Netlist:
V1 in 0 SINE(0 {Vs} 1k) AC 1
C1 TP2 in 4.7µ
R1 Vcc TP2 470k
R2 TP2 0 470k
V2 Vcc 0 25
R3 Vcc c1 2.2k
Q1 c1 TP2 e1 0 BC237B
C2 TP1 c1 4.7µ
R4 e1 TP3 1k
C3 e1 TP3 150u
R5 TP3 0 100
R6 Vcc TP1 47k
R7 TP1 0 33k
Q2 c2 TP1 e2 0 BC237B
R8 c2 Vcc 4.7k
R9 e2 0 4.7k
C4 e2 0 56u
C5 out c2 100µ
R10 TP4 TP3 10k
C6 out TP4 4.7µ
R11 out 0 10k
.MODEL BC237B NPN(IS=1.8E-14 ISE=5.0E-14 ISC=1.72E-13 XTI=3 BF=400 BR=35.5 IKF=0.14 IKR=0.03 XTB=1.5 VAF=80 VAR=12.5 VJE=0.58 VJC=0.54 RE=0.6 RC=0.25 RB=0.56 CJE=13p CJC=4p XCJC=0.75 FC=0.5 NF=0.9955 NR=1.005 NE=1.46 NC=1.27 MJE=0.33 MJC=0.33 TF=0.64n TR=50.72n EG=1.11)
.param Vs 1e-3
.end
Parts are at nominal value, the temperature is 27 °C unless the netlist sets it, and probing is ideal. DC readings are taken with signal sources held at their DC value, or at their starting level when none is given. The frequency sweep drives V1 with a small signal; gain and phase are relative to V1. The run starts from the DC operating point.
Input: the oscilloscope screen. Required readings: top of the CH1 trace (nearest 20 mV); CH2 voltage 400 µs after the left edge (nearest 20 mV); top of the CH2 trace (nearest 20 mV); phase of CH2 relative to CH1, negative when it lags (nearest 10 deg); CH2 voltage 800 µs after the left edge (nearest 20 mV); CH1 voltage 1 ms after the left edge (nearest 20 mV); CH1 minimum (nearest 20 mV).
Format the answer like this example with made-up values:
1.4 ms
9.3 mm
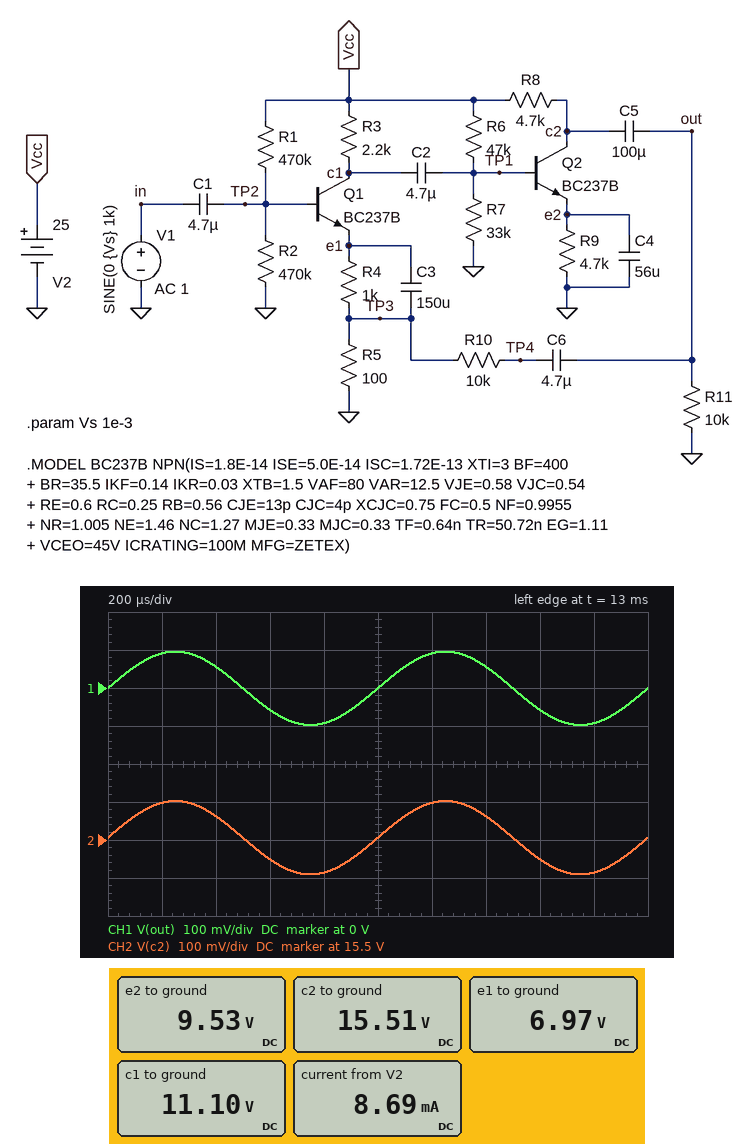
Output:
100 mV
15.56 V
15.60 V
0 deg
15.42 V
0 V
-100 mV
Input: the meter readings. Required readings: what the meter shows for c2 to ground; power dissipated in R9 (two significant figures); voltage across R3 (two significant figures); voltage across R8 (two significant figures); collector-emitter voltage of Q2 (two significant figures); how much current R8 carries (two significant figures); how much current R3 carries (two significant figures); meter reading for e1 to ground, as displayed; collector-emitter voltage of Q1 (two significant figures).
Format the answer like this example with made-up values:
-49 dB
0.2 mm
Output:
15.51 V
19 mW
14 V
9.5 V
6.0 V
2.0 mA
6.3 mA
6.97 V
4.1 V
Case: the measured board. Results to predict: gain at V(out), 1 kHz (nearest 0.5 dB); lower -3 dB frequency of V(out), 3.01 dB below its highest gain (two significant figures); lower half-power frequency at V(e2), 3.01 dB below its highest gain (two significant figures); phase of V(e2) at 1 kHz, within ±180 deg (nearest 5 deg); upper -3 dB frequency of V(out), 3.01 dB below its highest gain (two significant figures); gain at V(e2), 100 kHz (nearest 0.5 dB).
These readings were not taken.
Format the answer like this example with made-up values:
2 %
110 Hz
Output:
39.5 dB
7.9 Hz
7.2 Hz
90 deg
14 Hz
-59.0 dB
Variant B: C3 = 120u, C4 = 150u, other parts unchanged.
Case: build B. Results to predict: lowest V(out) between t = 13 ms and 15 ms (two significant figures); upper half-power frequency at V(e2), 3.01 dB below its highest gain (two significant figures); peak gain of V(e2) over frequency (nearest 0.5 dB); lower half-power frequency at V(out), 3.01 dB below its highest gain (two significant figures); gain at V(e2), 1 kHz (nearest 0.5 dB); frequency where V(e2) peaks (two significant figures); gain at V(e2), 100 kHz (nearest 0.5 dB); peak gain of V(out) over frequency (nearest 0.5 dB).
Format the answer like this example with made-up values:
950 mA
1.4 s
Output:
-97 mV
7.1 Hz
33.5 dB
6.2 Hz
-27.5 dB
6.6 Hz
-67.5 dB
57.5 dB
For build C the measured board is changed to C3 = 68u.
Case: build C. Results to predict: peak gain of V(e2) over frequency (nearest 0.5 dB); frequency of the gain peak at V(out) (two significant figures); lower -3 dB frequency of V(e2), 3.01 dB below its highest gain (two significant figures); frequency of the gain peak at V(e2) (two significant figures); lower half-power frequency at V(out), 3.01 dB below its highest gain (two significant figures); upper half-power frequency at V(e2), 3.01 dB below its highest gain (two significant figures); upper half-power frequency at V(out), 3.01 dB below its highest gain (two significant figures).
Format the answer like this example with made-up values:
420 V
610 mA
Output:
25.5 dB
14 Hz
10 Hz
13 Hz
11 Hz
16 Hz
19 Hz
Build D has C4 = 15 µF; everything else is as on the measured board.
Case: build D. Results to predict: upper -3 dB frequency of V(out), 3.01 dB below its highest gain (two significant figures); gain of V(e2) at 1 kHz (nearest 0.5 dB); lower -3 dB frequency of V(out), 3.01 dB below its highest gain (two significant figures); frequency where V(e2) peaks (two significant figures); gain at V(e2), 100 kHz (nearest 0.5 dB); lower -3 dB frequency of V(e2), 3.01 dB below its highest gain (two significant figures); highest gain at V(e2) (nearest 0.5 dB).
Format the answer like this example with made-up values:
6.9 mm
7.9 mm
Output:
7.4 MHz
-7.5 dB
16 Hz
17 Hz
-47.5 dB
9.1 Hz
25.5 dB
